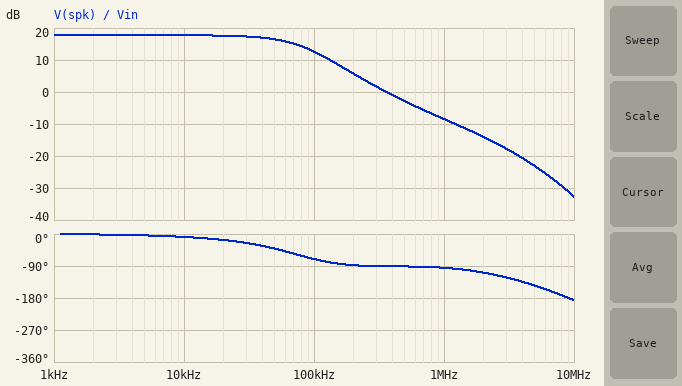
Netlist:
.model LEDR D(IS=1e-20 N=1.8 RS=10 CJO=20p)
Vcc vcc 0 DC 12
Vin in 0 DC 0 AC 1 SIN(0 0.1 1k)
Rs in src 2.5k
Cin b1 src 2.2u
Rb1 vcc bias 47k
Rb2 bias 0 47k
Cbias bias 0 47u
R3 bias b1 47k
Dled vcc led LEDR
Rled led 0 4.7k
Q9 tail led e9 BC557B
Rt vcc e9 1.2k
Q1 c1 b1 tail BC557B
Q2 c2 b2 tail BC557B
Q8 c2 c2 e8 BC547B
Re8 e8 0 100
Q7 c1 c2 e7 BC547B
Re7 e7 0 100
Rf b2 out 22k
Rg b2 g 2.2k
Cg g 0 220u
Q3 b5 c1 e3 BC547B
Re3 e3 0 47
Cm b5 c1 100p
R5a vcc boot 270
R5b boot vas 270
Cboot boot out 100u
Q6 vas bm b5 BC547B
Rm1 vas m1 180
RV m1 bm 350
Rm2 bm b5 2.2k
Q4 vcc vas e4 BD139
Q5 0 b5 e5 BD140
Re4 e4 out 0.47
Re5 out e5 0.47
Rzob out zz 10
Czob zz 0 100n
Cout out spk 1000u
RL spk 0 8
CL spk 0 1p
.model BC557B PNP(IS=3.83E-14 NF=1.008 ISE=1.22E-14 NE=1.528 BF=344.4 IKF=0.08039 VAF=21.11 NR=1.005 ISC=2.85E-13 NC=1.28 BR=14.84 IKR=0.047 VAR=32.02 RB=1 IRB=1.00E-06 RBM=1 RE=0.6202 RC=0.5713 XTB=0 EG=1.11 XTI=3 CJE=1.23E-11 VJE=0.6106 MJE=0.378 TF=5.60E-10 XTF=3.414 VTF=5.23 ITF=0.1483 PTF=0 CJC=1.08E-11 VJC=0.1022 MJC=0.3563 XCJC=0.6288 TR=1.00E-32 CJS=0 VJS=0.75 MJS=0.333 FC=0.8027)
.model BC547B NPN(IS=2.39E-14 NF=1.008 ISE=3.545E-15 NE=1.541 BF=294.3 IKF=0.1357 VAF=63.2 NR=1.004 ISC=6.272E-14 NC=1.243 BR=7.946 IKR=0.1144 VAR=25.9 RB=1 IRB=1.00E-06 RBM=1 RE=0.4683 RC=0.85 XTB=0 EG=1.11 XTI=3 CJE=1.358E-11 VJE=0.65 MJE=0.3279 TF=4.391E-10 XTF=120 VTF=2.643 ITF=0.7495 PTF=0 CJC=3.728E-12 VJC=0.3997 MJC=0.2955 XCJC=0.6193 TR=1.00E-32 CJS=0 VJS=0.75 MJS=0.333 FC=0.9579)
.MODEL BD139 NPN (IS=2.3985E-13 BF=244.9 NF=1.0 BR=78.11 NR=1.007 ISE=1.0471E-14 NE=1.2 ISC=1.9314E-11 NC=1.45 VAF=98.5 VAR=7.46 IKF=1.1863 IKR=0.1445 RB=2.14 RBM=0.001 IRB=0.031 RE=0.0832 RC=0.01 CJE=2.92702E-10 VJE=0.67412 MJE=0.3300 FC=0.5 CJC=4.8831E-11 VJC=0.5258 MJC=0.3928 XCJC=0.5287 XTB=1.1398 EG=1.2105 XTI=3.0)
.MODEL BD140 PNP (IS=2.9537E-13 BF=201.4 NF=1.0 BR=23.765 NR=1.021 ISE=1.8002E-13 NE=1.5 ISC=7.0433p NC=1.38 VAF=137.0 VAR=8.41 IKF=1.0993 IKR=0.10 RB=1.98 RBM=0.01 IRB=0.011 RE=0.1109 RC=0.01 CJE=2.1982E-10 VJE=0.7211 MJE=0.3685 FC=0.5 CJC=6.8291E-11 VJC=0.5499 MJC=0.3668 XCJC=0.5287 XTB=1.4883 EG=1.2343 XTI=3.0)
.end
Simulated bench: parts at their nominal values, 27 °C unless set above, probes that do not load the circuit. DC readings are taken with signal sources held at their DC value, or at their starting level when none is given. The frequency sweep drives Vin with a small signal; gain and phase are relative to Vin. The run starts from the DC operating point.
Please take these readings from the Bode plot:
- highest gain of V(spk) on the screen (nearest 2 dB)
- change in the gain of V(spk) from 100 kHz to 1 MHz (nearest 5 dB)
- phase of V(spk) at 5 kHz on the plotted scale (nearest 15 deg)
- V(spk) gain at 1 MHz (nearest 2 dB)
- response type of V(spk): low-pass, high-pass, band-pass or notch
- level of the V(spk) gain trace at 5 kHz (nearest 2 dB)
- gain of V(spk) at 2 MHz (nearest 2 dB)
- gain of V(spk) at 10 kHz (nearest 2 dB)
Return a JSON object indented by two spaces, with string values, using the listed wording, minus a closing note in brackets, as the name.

{
  "highest gain of V(spk) on the screen": "18 dB",
  "change in the gain of V(spk) from 100 kHz to 1 MHz": "-20 dB",
  "phase of V(spk) at 5 kHz on the plotted scale": "0 deg",
  "V(spk) gain at 1 MHz": "-8 dB",
  "response type of V(spk): low-pass, high-pass, band-pass or notch": "low-pass",
  "level of the V(spk) gain trace at 5 kHz": "18 dB",
  "gain of V(spk) at 2 MHz": "-14 dB",
  "gain of V(spk) at 10 kHz": "18 dB"
}
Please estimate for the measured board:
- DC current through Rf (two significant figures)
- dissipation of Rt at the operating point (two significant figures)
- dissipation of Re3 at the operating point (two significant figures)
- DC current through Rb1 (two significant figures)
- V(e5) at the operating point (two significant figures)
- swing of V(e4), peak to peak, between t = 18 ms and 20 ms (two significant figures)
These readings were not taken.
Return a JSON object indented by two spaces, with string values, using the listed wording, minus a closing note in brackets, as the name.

{
  "DC current through Rf": "1.2 µA",
  "dissipation of Rt at the operating point": "1.3 mW",
  "dissipation of Re3 at the operating point": "4.9 mW",
  "DC current through Rb1": "130 µA",
  "V(e5) at the operating point": "6.1 V",
  "swing of V(e4), peak to peak, between t = 18 ms and 20 ms": "2.1 V"
}
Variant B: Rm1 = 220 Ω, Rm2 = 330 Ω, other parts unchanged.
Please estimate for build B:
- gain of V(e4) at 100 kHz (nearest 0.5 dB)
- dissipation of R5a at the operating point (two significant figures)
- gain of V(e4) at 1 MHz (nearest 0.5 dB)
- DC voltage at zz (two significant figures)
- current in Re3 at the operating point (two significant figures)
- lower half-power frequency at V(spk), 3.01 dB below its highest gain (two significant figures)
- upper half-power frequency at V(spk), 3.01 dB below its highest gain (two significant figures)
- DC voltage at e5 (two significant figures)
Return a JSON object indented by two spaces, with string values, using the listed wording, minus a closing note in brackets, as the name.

{
  "gain of V(e4) at 100 kHz": "20.5 dB",
  "dissipation of R5a at the operating point": "23 mW",
  "gain of V(e4) at 1 MHz": "22.5 dB",
  "DC voltage at zz": "6.1 V",
  "current in Re3 at the operating point": "9.6 mA",
  "lower half-power frequency at V(spk), 3.01 dB below its highest gain": "54 Hz",
  "upper half-power frequency at V(spk), 3.01 dB below its highest gain": "2.1 MHz",
  "DC voltage at e5": "5.9 V"
}
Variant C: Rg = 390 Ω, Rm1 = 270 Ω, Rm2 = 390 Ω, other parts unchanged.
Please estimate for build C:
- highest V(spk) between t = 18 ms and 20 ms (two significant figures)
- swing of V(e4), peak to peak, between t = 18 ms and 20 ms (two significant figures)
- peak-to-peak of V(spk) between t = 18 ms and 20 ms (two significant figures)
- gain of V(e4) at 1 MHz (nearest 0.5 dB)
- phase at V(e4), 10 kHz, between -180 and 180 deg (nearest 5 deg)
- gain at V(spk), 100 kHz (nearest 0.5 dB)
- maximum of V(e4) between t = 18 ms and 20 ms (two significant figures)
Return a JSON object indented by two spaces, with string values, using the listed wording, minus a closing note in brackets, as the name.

{
  "highest V(spk) between t = 18 ms and 20 ms": "5.2 V",
  "swing of V(e4), peak to peak, between t = 18 ms and 20 ms": "9.8 V",
  "peak-to-peak of V(spk) between t = 18 ms and 20 ms": "9.5 V",
  "gain of V(e4) at 1 MHz": "26.5 dB",
  "phase at V(e4), 10 kHz, between -180 and 180 deg": "0 deg",
  "gain at V(spk), 100 kHz": "34.5 dB",
  "maximum of V(e4) between t = 18 ms and 20 ms": "12 V"
}
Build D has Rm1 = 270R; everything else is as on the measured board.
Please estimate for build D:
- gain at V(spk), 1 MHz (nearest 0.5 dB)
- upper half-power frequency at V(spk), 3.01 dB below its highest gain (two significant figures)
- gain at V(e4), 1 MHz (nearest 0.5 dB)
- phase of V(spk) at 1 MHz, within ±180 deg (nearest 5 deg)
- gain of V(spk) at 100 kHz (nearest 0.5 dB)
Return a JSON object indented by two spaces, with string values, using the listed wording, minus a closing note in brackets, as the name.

{
  "gain at V(spk), 1 MHz": "-8.0 dB",
  "upper half-power frequency at V(spk), 3.01 dB below its highest gain": "81 kHz",
  "gain at V(e4), 1 MHz": "-7.5 dB",
  "phase of V(spk) at 1 MHz, within ±180 deg": "-100 deg",
  "gain of V(spk) at 100 kHz": "13.5 dB"
}
